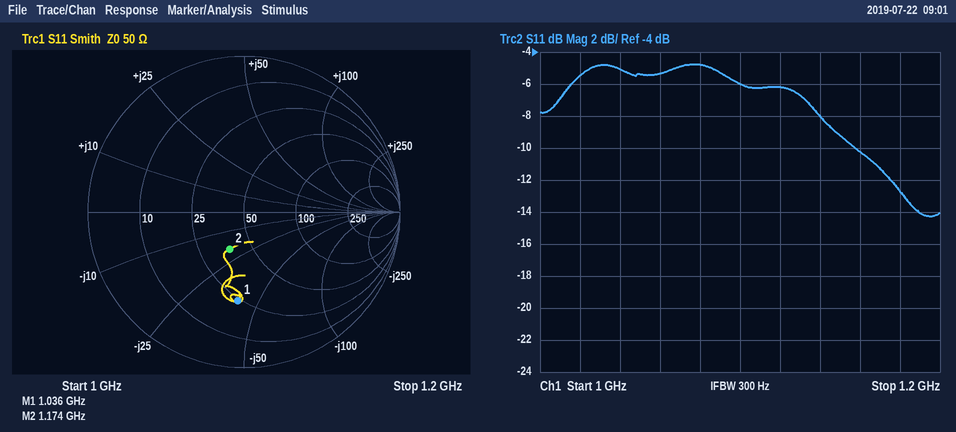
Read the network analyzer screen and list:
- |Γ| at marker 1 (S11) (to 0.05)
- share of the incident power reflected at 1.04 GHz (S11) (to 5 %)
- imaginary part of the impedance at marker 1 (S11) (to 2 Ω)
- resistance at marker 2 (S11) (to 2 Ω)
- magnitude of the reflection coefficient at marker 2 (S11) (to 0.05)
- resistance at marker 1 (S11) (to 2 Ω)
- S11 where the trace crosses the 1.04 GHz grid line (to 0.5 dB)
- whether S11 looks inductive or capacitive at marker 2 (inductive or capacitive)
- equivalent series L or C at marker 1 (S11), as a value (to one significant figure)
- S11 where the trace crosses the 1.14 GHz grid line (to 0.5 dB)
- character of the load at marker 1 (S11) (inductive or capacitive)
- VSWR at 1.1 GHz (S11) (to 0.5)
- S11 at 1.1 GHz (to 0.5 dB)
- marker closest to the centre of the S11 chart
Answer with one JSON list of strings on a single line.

["0.55", "30 %", "-40 Ω", "38 Ω", "0.25", "24 Ω", "-5.0 dB", "capacitive", "4 pF", "-8.0 dB", "capacitive", "3.0", "-6.0 dB", "marker 2"]
